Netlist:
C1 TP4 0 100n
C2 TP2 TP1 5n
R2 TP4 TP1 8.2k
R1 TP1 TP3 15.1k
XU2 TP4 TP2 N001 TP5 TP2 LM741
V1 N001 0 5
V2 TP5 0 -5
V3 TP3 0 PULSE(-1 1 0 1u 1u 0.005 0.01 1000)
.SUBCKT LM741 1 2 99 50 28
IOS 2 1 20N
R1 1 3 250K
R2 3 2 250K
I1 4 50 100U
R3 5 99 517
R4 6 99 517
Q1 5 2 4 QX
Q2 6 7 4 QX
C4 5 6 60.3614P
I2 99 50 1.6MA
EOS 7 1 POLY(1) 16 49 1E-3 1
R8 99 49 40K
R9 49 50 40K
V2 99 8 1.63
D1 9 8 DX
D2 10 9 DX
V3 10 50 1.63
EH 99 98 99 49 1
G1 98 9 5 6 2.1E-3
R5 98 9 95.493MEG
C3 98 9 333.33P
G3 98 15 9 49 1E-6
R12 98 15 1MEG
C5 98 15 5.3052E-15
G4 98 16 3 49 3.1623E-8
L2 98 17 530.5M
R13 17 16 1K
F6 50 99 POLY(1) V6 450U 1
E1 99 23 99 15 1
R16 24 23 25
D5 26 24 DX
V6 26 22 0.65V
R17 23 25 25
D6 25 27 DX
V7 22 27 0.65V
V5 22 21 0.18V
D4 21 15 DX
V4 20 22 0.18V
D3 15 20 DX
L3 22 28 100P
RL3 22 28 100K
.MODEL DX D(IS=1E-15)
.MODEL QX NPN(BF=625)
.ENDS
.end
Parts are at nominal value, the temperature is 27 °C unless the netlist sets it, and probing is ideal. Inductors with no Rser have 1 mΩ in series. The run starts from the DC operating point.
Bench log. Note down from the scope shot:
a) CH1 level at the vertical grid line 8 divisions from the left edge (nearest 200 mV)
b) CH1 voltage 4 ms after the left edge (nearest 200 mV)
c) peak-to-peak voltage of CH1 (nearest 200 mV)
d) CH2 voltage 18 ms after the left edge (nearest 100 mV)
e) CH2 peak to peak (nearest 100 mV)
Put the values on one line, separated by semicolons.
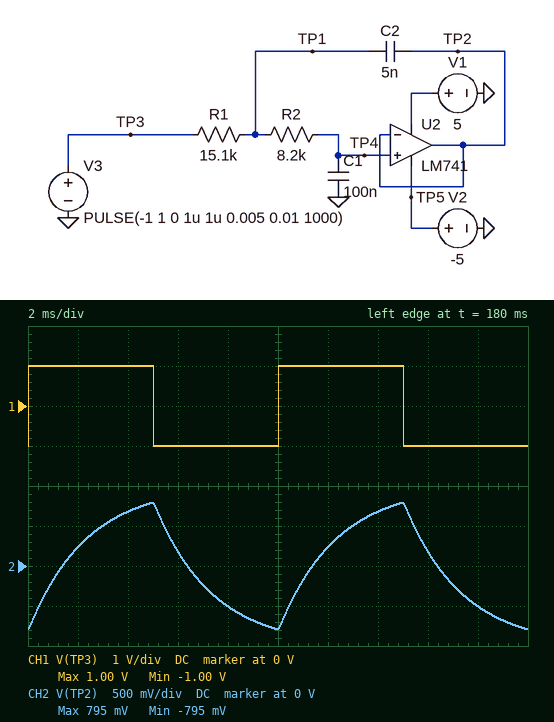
-1.0 V; 1.0 V; 2.0 V; -500 mV; 1.6 V
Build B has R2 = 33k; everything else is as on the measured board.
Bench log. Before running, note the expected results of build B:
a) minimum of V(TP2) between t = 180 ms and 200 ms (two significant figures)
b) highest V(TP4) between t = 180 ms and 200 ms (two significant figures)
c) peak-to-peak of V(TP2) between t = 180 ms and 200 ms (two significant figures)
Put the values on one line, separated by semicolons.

-480 mV; 470 mV; 950 mV
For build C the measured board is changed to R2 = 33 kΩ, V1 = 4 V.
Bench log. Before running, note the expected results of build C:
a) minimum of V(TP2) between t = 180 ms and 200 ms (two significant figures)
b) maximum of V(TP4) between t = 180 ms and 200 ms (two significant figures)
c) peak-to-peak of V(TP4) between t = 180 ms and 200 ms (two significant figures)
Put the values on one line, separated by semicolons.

-480 mV; 470 mV; 950 mV
